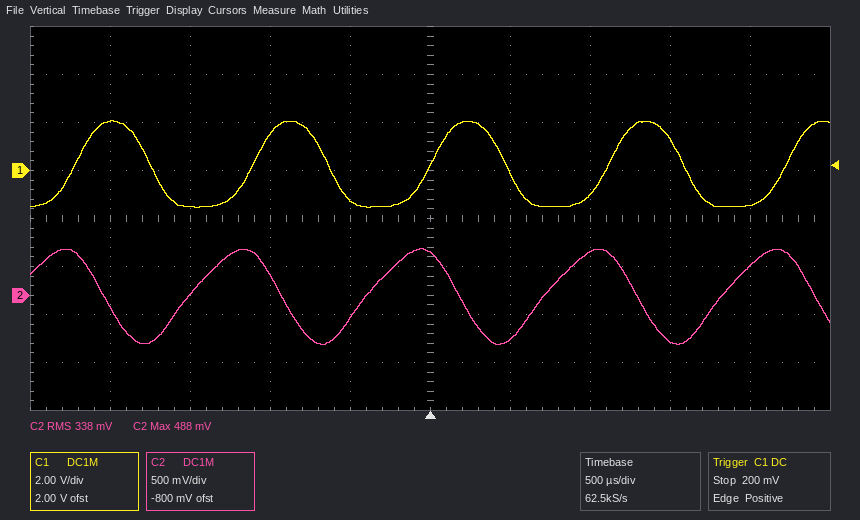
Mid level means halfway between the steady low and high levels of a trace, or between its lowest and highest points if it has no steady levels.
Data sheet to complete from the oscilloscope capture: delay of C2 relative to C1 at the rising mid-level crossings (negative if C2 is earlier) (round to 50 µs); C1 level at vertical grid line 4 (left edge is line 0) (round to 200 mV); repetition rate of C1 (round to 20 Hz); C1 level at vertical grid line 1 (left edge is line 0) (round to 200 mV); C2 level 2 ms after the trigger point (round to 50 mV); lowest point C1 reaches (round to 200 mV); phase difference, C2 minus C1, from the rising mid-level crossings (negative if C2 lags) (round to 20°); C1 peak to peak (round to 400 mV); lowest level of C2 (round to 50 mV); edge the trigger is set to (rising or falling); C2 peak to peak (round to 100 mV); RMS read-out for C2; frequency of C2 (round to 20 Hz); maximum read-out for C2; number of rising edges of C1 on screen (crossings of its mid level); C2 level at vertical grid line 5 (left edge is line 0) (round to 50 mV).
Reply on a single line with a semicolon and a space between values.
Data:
-400 µs; -1.2 V; 900 Hz; 2.0 V; 300 mV; -1.6 V; +140°; 3.6 V; -500 mV; rising; 1.00 V; 338 mV; 900 Hz; 488 mV; 5; 450 mV
